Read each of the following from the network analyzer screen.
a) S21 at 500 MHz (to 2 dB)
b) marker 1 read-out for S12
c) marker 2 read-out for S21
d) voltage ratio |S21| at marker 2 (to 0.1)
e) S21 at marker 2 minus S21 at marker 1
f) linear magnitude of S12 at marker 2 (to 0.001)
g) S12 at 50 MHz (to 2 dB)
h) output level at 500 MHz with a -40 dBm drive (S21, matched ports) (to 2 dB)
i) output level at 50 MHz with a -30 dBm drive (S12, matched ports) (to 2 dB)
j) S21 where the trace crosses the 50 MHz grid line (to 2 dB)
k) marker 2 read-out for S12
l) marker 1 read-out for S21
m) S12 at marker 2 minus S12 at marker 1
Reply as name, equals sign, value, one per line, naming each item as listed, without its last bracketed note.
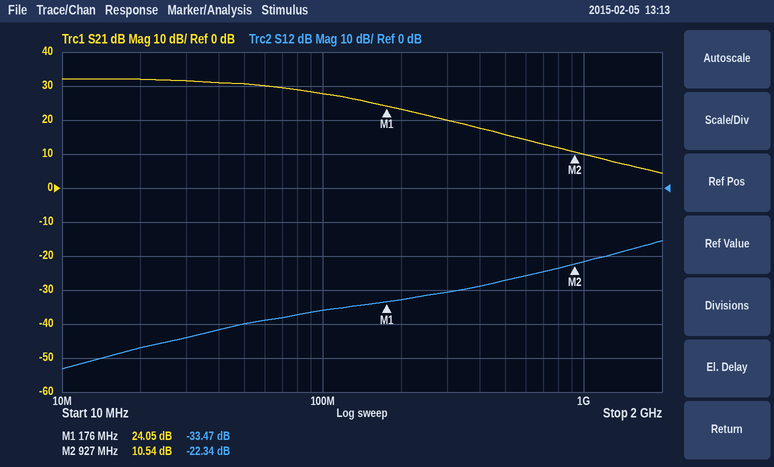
S21 at 500 MHz = 16 dB
marker 1 read-out for S12 = -33.47 dB
marker 2 read-out for S21 = 10.54 dB
voltage ratio |S21| at marker 2 = 3.4
S21 at marker 2 minus S21 at marker 1 = -13.51 dB
linear magnitude of S12 at marker 2 = 0.076
S12 at 50 MHz = -40 dB
output level at 500 MHz with a -40 dBm drive (S21, matched ports) = -24 dBm
output level at 50 MHz with a -30 dBm drive (S12, matched ports) = -70 dBm
S21 where the trace crosses the 50 MHz grid line = 30 dB
marker 2 read-out for S12 = -22.34 dB
marker 1 read-out for S21 = 24.05 dB
S12 at marker 2 minus S12 at marker 1 = 11.13 dB
